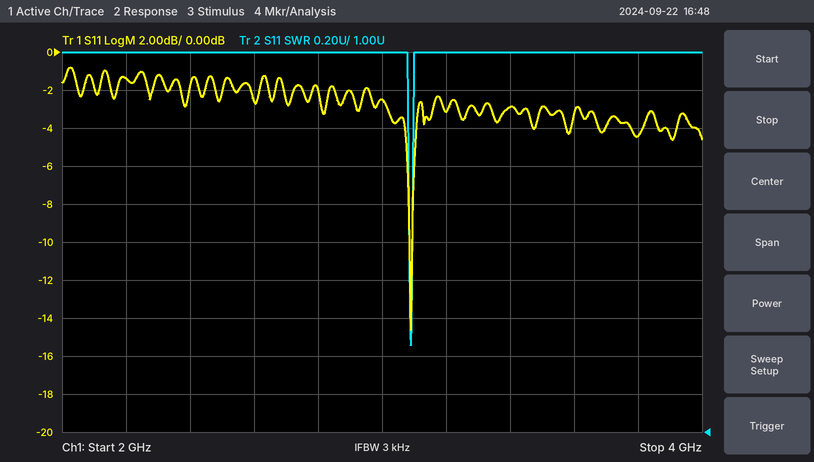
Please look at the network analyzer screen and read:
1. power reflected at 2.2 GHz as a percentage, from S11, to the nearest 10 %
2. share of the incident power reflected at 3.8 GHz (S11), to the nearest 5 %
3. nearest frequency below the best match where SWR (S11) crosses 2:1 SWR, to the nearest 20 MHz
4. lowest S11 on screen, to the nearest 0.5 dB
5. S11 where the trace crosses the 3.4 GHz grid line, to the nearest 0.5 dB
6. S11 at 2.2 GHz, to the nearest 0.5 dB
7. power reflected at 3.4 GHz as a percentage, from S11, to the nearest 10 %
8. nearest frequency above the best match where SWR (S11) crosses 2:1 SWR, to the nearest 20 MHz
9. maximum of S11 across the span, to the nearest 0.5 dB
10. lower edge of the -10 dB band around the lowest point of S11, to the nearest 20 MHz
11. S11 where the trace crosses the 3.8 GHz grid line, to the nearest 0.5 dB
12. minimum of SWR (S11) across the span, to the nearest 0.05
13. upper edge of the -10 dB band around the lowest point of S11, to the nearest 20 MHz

70 %
35 %
3.08 GHz
-14.5 dB
-3.0 dB
-1.5 dB
50 %
3.10 GHz
-1.0 dB
3.08 GHz
-4.5 dB
1.45
3.10 GHz
